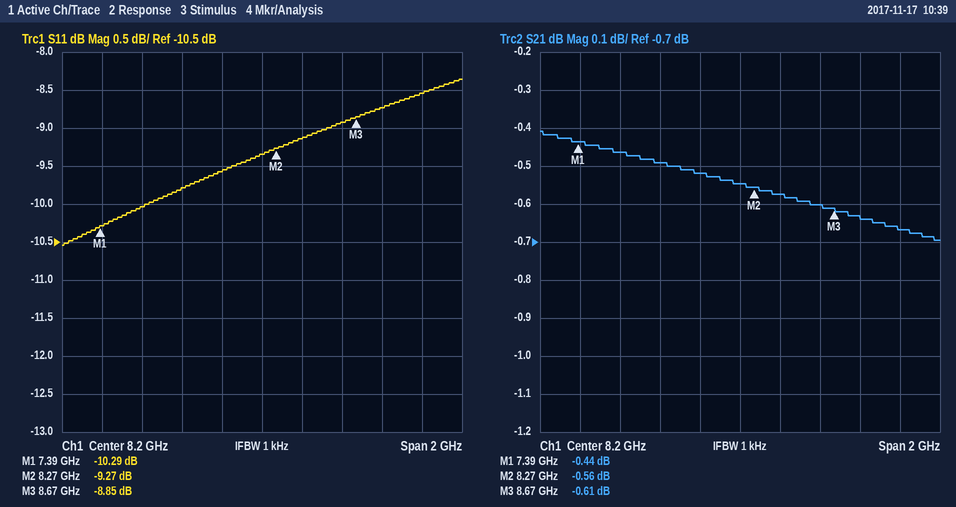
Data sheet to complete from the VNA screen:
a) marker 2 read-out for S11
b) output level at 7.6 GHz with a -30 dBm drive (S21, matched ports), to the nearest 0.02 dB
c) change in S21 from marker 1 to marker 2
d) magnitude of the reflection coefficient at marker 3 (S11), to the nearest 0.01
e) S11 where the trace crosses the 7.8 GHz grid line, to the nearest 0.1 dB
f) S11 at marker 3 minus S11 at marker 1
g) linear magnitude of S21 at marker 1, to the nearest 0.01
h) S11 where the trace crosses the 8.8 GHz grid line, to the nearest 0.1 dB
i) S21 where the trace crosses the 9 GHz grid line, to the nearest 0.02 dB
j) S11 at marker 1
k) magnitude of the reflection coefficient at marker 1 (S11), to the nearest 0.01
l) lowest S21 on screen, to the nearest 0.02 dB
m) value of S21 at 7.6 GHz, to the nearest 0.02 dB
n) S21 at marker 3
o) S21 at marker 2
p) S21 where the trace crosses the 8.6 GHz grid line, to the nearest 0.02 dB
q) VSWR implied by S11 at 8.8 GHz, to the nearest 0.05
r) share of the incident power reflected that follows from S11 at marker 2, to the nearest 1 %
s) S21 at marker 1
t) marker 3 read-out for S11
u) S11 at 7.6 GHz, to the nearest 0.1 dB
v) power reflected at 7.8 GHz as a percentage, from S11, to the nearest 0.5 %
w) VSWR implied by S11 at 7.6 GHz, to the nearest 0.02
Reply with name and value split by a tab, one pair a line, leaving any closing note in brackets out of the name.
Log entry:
marker 2 read-out for S11	-9.27 dB
output level at 7.6 GHz with a -30 dBm drive (S21, matched ports), to the nearest 0.02 dB	-30.46 dBm
change in S21 from marker 1 to marker 2	-0.12 dB
magnitude of the reflection coefficient at marker 3 (S11), to the nearest 0.01	0.36
S11 where the trace crosses the 7.8 GHz grid line, to the nearest 0.1 dB	-9.8 dB
S11 at marker 3 minus S11 at marker 1	1.44 dB
linear magnitude of S21 at marker 1, to the nearest 0.01	0.95
S11 where the trace crosses the 8.8 GHz grid line, to the nearest 0.1 dB	-8.7 dB
S21 where the trace crosses the 9 GHz grid line, to the nearest 0.02 dB	-0.66 dB
S11 at marker 1	-10.29 dB
magnitude of the reflection coefficient at marker 1 (S11), to the nearest 0.01	0.31
lowest S21 on screen, to the nearest 0.02 dB	-0.70 dB
value of S21 at 7.6 GHz, to the nearest 0.02 dB	-0.46 dB
S21 at marker 3	-0.61 dB
S21 at marker 2	-0.56 dB
S21 where the trace crosses the 8.6 GHz grid line, to the nearest 0.02 dB	-0.60 dB
VSWR implied by S11 at 8.8 GHz, to the nearest 0.05	2.15
share of the incident power reflected that follows from S11 at marker 2, to the nearest 1 %	12 %
S21 at marker 1	-0.44 dB
marker 3 read-out for S11	-8.85 dB
S11 at 7.6 GHz, to the nearest 0.1 dB	-10.0 dB
power reflected at 7.8 GHz as a percentage, from S11, to the nearest 0.5 %	10.5 %
VSWR implied by S11 at 7.6 GHz, to the nearest 0.02	1.92
